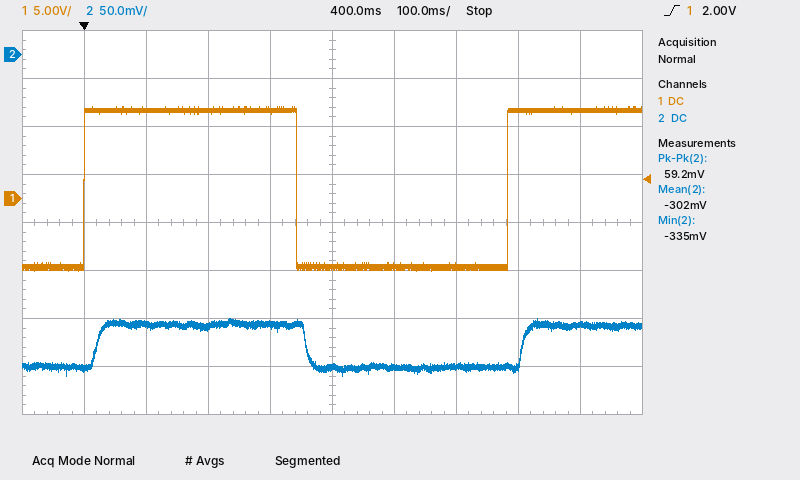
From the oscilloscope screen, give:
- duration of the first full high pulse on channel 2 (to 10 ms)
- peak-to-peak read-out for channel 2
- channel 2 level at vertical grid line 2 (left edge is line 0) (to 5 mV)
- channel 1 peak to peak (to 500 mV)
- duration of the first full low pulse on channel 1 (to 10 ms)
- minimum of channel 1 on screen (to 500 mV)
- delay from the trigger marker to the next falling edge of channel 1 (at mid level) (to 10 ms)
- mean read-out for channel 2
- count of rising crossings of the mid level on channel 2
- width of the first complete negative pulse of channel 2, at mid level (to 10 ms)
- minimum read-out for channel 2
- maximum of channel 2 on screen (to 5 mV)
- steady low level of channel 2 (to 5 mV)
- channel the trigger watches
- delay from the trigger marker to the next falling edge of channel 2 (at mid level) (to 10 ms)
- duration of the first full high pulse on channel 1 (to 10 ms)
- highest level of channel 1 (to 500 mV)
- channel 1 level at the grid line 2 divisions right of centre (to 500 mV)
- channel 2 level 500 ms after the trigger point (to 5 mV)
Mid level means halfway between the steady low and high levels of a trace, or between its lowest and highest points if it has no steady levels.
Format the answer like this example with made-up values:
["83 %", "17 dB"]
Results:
["340 ms", "59.2 mV", "-280 mV", "17.0 V", "340 ms", "-7.5 V", "340 ms", "-302 mV", "2", "350 ms", "-335 mV", "-275 mV", "-325 mV", "channel 1", "360 ms", "340 ms", "9.5 V", "-7.0 V", "-325 mV"]
